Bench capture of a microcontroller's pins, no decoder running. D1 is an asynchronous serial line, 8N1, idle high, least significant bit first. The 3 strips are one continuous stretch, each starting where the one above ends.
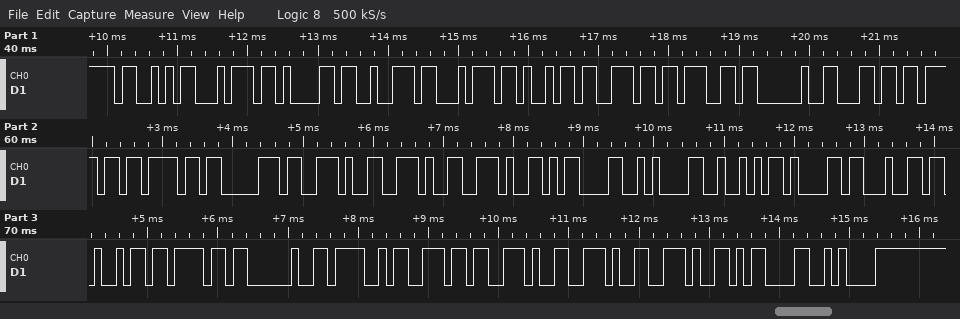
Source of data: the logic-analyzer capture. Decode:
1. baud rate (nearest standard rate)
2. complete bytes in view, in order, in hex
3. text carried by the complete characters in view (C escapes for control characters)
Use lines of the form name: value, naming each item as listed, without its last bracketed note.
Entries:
baud rate: 9600 baud
complete bytes in view, in order, in hex: 0x53 0x74 0x61 0x72 0x74 0x69 0x6E 0x67 0x20 0x6C 0x6F 0x6F 0x70 0x2E 0x2E 0x2E 0x0D 0x0A 0x52 0x61 0x64 0x69 0x6F 0x20 0x4F 0x6E 0x2E 0x2E 0x2E 0x0D 0x0A
text carried by the complete characters in view: "Starting loop...\r\nRadio On...\r\n"
